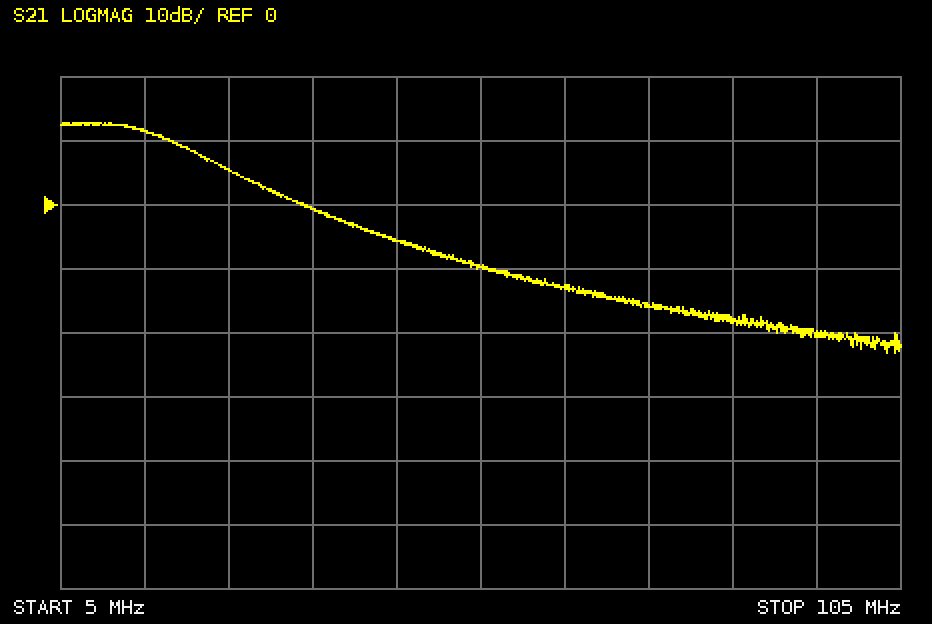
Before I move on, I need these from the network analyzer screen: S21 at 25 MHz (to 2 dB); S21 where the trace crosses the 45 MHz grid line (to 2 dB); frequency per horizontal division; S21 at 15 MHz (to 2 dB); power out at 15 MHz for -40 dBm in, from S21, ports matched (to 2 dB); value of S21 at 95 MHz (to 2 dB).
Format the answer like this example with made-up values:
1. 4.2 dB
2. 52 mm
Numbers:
1. 6 dB
2. -6 dB
3. 10 MHz
4. 12 dB
5. -28 dBm
6. -20 dB
